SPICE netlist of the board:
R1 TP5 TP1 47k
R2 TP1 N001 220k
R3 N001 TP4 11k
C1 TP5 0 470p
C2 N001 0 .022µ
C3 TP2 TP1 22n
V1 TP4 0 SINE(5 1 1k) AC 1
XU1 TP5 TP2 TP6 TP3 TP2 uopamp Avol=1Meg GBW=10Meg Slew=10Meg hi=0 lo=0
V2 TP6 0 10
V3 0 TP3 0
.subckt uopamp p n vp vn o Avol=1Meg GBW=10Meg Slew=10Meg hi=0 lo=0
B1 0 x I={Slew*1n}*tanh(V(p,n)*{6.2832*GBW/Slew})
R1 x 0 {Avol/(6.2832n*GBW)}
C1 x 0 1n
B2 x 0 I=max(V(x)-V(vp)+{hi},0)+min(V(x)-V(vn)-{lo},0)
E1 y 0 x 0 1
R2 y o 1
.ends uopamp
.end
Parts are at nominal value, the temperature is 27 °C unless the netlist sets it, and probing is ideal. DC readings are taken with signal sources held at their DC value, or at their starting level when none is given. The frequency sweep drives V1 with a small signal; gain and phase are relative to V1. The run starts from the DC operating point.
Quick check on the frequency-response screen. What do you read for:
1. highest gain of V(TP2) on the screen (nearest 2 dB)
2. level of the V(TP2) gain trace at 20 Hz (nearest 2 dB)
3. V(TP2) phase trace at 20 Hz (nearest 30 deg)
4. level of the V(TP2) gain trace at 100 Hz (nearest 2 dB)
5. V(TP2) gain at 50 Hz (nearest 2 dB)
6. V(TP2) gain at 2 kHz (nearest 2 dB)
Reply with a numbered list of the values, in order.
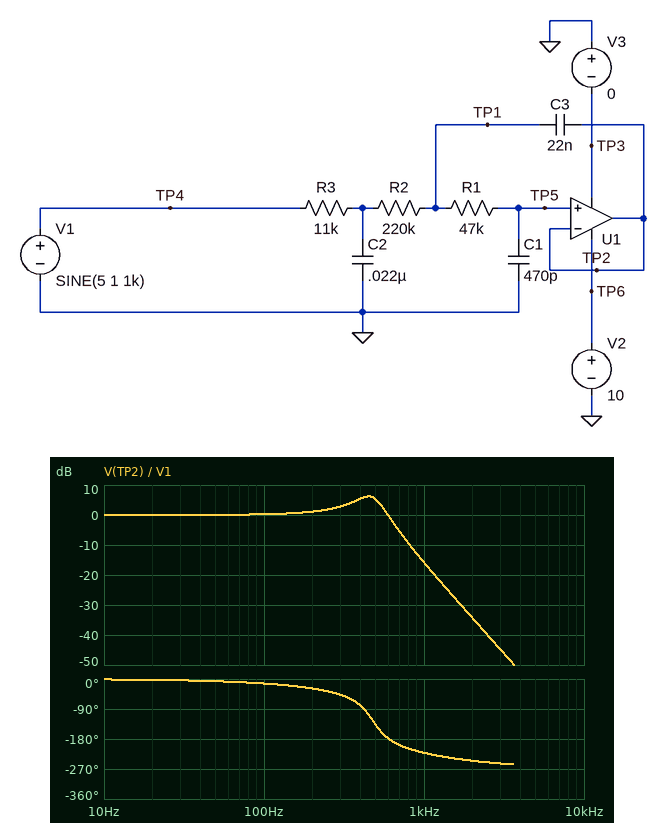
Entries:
1. 6 dB
2. 0 dB
3. 0 deg
4. 0 dB
5. 0 dB
6. -34 dB
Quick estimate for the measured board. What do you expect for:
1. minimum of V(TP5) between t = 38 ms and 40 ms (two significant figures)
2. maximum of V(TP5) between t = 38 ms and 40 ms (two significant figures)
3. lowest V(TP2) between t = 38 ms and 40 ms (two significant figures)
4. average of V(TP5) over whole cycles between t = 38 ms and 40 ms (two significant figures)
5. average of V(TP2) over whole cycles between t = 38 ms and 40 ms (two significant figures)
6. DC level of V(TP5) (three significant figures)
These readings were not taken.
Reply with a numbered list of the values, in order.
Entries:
1. 4.8 V
2. 5.2 V
3. 4.8 V
4. 5.0 V
5. 5.0 V
6. 5.00 V
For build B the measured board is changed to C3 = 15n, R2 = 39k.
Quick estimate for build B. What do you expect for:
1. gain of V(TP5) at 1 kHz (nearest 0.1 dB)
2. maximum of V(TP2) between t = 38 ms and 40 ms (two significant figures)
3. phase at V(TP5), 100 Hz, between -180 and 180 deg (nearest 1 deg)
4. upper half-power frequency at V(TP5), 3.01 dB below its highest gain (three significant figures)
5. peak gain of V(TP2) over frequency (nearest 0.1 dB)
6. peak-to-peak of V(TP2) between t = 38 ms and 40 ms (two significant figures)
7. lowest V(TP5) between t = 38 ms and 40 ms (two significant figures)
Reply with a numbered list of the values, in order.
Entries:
1. -0.3 dB
2. 6.0 V
3. -10 deg
4. 1.51 kHz
5. 0.3 dB
6. 1.9 V
7. 4.0 V
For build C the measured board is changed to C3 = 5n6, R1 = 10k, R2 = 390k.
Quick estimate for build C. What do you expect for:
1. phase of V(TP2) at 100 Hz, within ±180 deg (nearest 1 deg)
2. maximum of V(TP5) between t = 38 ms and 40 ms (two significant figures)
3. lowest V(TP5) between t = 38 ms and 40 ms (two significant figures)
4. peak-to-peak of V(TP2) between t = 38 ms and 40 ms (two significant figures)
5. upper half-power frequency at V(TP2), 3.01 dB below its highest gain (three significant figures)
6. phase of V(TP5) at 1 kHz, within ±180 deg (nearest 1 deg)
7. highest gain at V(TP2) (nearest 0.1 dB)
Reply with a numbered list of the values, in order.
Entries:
1. -16 deg
2. 5.4 V
3. 4.6 V
4. 820 mV
5. 534 Hz
6. -120 deg
7. 0 dB
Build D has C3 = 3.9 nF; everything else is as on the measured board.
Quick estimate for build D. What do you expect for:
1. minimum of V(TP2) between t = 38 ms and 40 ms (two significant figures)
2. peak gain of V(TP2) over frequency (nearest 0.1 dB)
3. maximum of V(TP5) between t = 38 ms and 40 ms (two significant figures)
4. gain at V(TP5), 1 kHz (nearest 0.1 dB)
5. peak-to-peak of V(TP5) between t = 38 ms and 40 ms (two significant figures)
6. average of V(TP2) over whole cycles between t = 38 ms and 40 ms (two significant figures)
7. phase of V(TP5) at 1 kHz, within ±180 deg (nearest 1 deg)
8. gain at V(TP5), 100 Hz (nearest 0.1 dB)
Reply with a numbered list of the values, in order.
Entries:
1. 4.4 V
2. 0 dB
3. 5.6 V
4. -3.8 dB
5. 1.3 V
6. 5.0 V
7. -129 deg
8. -0.1 dB
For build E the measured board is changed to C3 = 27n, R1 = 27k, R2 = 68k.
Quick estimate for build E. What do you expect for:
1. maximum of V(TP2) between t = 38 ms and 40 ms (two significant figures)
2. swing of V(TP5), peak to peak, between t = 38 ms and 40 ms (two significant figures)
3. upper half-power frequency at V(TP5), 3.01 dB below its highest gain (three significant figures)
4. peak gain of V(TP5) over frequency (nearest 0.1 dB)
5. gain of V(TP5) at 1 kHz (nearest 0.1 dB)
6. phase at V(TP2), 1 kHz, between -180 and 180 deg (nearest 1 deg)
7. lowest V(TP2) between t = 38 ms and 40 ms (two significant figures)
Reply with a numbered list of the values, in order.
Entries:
1. 6.5 V
2. 3.0 V
3. 1.13 kHz
4. 3.8 dB
5. 3.6 dB
6. -139 deg
7. 3.5 V
